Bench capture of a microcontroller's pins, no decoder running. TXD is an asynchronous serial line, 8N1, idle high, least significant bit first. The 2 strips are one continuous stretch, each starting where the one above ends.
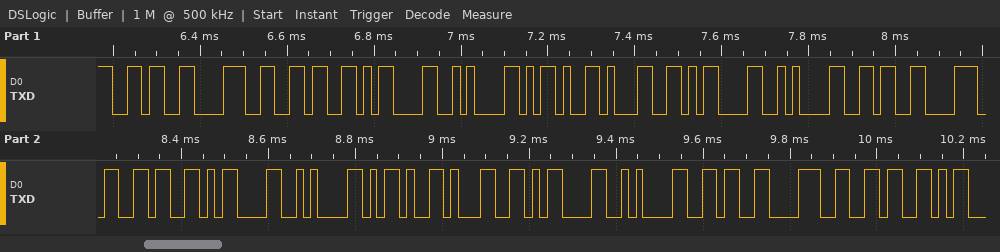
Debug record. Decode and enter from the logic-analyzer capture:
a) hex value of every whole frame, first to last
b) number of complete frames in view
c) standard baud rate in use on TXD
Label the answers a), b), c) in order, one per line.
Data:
a) 0x36 0x38 0x36 0x0D 0x0A 0x2D 0x31 0x0D 0x0A 0x36 0x38 0x36 0x0D 0x0A 0x2D 0x31 0x0D 0x0A 0x36 0x38 0x36
b) 21
c) 57600 baud
